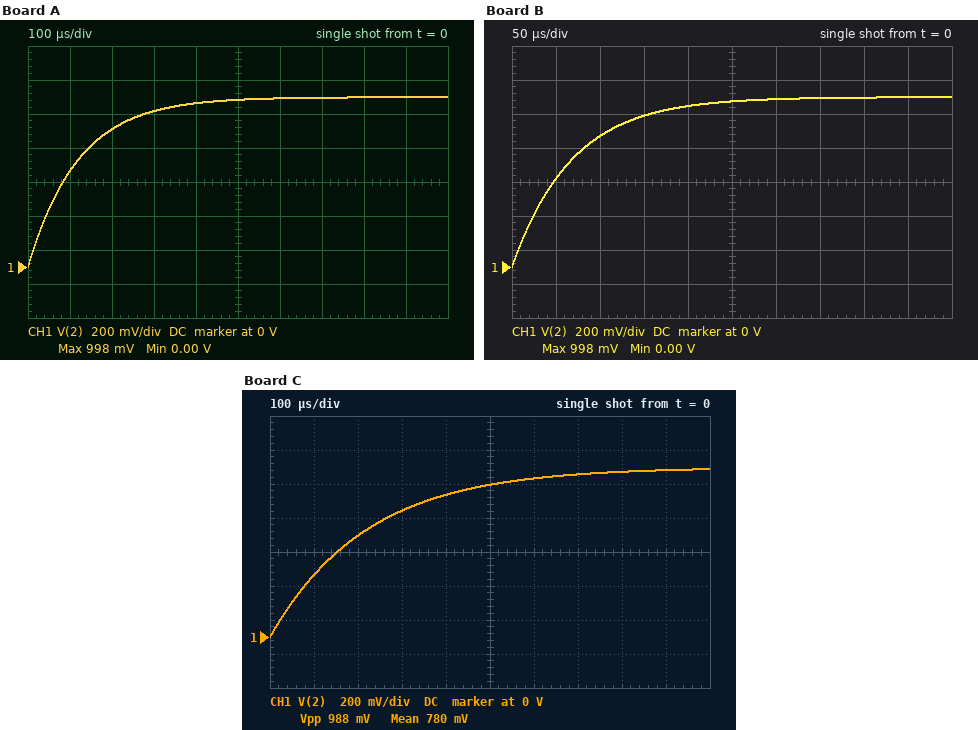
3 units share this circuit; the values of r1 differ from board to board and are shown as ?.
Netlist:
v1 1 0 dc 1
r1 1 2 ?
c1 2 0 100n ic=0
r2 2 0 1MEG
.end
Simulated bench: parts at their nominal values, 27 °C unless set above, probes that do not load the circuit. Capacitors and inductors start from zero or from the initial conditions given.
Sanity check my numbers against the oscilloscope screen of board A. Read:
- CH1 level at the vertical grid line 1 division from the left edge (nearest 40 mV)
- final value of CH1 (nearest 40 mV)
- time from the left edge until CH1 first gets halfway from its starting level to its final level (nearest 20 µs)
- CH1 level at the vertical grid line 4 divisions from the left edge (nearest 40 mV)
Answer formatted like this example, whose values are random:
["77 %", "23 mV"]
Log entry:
["560 mV", "1.00 V", "80 µs", "960 mV"]
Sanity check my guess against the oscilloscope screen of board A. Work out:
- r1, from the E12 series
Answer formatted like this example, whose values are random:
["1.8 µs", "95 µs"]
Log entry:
["1.2 kΩ"]
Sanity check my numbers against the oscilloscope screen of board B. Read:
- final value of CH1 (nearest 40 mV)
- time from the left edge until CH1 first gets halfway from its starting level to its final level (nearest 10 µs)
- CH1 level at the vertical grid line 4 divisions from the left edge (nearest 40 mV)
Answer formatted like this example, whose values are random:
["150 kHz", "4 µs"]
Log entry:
["1.00 V", "50 µs", "960 mV"]
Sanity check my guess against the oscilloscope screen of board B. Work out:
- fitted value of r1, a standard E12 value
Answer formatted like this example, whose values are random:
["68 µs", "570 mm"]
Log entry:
["680 Ω"]
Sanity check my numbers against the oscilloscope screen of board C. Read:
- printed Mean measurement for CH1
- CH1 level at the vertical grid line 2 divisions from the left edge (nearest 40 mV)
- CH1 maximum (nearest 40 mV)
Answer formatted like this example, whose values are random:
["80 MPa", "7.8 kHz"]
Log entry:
["780 mV", "600 mV", "1.00 V"]
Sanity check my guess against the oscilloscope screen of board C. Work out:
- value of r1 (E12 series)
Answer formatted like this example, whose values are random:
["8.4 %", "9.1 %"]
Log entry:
["2.2 kΩ"]
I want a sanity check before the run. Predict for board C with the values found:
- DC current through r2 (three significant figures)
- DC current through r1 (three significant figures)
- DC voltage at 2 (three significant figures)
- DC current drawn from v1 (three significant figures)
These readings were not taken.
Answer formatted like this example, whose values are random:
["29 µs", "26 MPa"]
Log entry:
["998 nA", "998 nA", "998 mV", "998 nA"]
